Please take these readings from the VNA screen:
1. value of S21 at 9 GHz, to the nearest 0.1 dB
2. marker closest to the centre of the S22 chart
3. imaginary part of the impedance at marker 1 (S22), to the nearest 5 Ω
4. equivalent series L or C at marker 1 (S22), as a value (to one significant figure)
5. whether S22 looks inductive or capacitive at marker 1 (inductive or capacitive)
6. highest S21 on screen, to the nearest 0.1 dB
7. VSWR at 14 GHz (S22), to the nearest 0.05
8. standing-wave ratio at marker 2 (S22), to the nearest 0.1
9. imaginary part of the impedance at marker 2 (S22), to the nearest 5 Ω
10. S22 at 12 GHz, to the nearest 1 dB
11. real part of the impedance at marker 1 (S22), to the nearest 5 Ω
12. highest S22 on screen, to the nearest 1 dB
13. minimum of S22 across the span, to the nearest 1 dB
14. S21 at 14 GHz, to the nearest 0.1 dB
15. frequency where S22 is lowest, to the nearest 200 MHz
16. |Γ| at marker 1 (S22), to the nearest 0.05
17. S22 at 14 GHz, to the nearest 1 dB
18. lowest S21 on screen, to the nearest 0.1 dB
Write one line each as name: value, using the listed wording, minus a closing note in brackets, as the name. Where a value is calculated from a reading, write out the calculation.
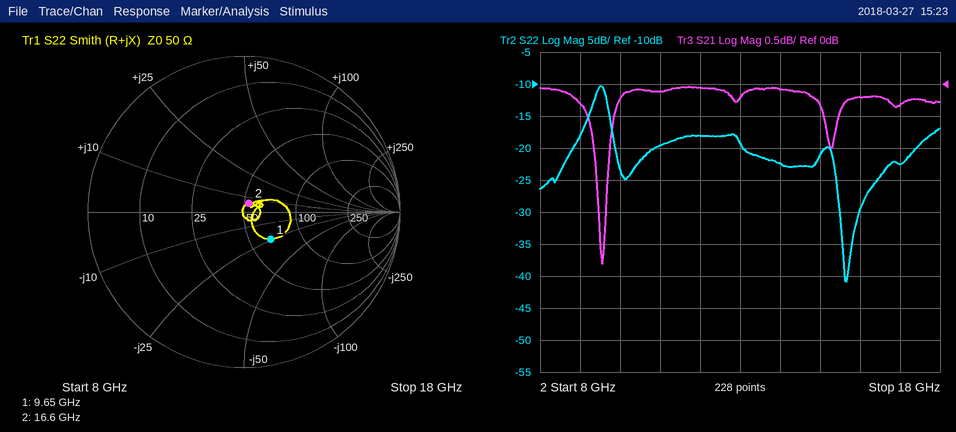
value of S21 at 9 GHz, to the nearest 0.1 dB: -0.3 dB
marker closest to the centre of the S22 chart: marker 2
imaginary part of the impedance at marker 1 (S22), to the nearest 5 Ω: -25 Ω
equivalent series L or C at marker 1 (S22), as a value: C = 1/(2π × 9.65 GHz × 25 Ω) ≈ 660 fF, so 700 fF to one significant figure
whether S22 looks inductive or capacitive at marker 1: capacitive
highest S21 on screen, to the nearest 0.1 dB: 0.0 dB
VSWR at 14 GHz (S22), to the nearest 0.05: |Γ| = 10^(-22/20) = 0.0794; VSWR = (1 + 0.0794)/(1 − 0.0794) ≈ 1.17, so 1.15 to the nearest 0.05
standing-wave ratio at marker 2 (S22), to the nearest 0.1: 1.1
imaginary part of the impedance at marker 2 (S22), to the nearest 5 Ω: +5 Ω
S22 at 12 GHz, to the nearest 1 dB: -18 dB
real part of the impedance at marker 1 (S22), to the nearest 5 Ω: 65 Ω
highest S22 on screen, to the nearest 1 dB: -10 dB
minimum of S22 across the span, to the nearest 1 dB: -41 dB
S21 at 14 GHz, to the nearest 0.1 dB: -0.1 dB
frequency where S22 is lowest, to the nearest 200 MHz: 15.6 GHz
|Γ| at marker 1 (S22), to the nearest 0.05: 0.25
S22 at 14 GHz, to the nearest 1 dB: -22 dB
lowest S21 on screen, to the nearest 0.1 dB: -2.8 dB
